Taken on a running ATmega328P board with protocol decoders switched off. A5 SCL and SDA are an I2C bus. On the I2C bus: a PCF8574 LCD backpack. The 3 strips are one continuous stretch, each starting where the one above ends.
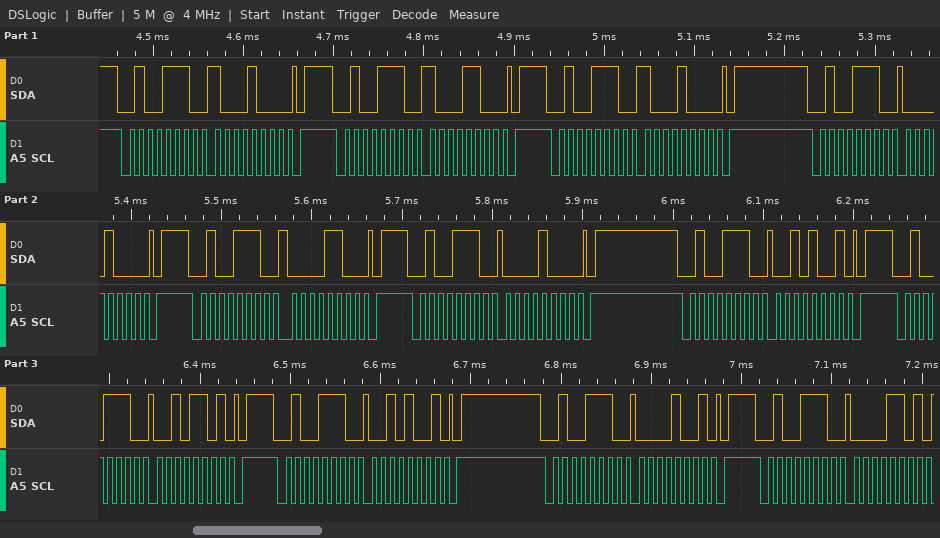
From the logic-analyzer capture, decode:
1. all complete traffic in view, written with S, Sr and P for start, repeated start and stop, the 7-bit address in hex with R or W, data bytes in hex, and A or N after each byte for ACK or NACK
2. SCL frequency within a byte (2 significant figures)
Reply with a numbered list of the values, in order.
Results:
1. S 27W A 88 A P S 27W A 8C A P S 27W A 88 A P S 27W A 08 A P S 27W A 0C A P S 27W A 08 A P S 27W A 29 A P S 27W A 2D A P S 27W A 29 A P S 27W A 09 A P S 27W A 0D A
2. 100 kHz
